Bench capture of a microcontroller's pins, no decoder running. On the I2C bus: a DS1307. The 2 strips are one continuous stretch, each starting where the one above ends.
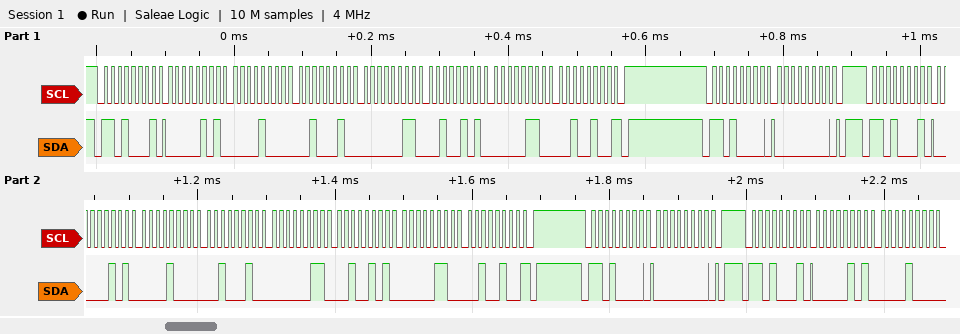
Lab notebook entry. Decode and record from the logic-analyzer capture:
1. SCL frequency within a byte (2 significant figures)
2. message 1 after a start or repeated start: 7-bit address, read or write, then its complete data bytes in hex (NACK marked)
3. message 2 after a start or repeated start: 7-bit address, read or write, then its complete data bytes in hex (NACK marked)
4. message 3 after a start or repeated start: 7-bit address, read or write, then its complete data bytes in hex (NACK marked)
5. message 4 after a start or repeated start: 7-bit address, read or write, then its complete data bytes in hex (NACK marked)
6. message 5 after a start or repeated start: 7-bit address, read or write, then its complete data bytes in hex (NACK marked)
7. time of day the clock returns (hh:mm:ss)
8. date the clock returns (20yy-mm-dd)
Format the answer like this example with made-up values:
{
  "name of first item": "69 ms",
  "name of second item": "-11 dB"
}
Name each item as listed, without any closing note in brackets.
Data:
{
  "SCL frequency within a byte": "100 kHz",
  "message 1 after a start or repeated start: 7-bit address, read or write, then its complete data bytes in hex": "0x68 read: 05 08 22 03 25 06 24 NACK",
  "message 2 after a start or repeated start: 7-bit address, read or write, then its complete data bytes in hex": "0x68 write: 00",
  "message 3 after a start or repeated start: 7-bit address, read or write, then its complete data bytes in hex": "0x68 read: 05 08 22 03 25 06 24 NACK",
  "message 4 after a start or repeated start: 7-bit address, read or write, then its complete data bytes in hex": "0x68 write: 00",
  "message 5 after a start or repeated start: 7-bit address, read or write, then its complete data bytes in hex": "0x68 read: 05 08",
  "time of day the clock returns": "22:08:05",
  "date the clock returns": "2024-06-25"
}
